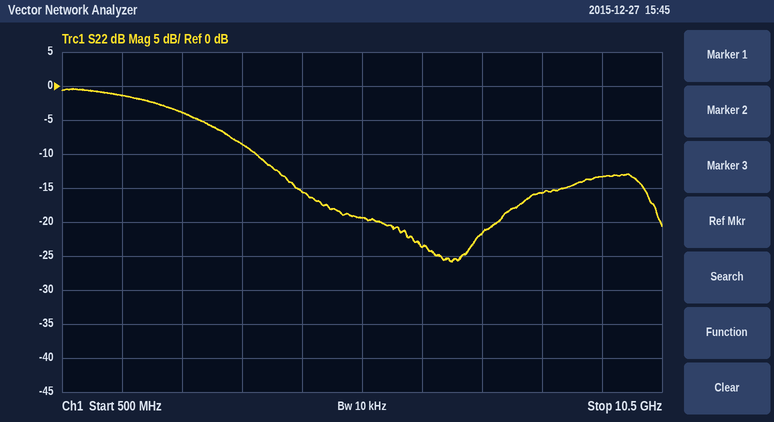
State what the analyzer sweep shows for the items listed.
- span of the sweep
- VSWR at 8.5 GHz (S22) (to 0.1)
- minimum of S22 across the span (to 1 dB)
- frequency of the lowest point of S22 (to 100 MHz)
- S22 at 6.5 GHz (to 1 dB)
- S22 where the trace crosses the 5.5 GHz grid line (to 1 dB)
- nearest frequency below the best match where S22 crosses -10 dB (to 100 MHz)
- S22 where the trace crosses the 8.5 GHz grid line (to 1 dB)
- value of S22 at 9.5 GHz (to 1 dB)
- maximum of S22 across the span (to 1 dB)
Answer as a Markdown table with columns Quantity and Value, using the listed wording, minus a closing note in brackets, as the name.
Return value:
| Quantity | Value |
|---|---|
| span of the sweep | 10 GHz |
| VSWR at 8.5 GHz (S22) | 1.4 |
| minimum of S22 across the span | -26 dB |
| frequency of the lowest point of S22 | 7.0 GHz |
| S22 at 6.5 GHz | -24 dB |
| S22 where the trace crosses the 5.5 GHz grid line | -19 dB |
| nearest frequency below the best match where S22 crosses -10 dB | 3.7 GHz |
| S22 where the trace crosses the 8.5 GHz grid line | -16 dB |
| value of S22 at 9.5 GHz | -13 dB |
| maximum of S22 across the span | 0 dB |
